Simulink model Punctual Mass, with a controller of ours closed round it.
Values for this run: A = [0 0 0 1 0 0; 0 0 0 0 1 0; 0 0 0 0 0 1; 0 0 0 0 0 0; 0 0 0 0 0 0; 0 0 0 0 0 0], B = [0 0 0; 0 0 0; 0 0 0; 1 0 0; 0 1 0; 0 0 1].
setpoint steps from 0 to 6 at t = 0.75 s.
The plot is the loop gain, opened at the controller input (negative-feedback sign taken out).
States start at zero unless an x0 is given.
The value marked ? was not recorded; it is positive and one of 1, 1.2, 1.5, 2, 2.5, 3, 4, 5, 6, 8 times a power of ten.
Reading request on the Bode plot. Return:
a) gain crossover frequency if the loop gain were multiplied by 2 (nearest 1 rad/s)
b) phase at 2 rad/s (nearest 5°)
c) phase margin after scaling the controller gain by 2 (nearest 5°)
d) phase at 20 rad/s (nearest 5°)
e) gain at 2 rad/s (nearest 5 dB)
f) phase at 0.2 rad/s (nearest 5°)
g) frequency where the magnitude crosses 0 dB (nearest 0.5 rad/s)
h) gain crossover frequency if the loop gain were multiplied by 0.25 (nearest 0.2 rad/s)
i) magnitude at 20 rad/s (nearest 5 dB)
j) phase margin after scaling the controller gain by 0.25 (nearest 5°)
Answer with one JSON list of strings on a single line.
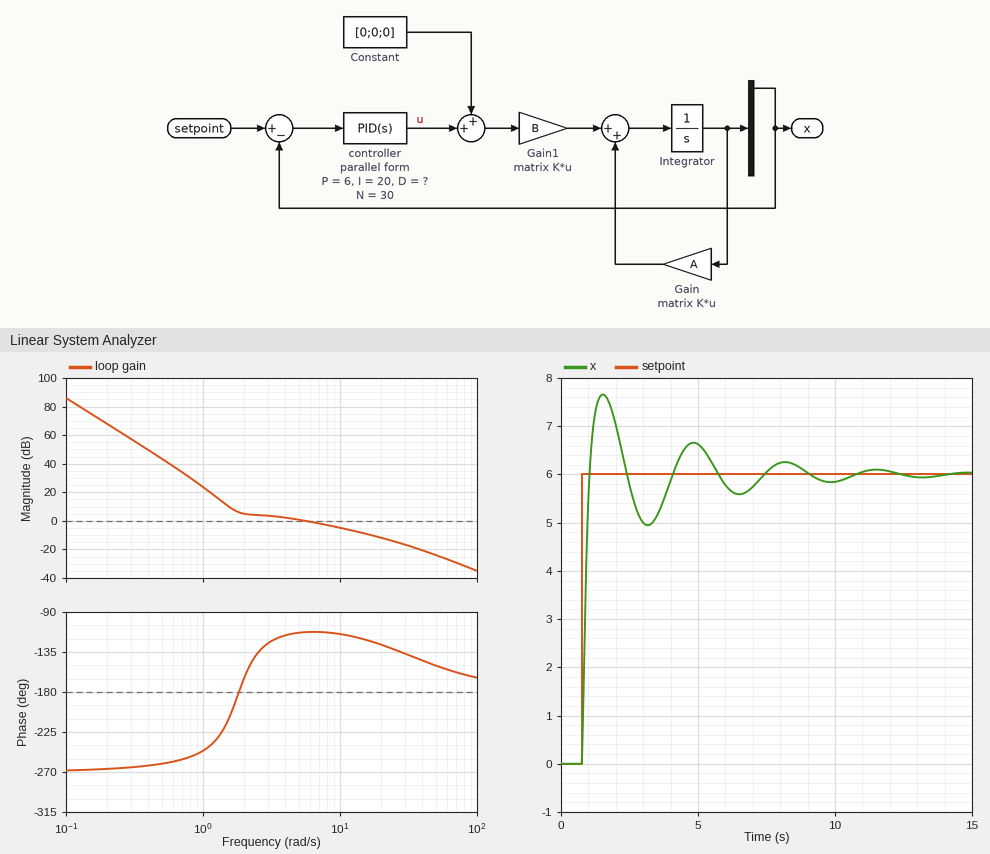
["11 rad/s", "-165°", "65°", "-125°", "5 dB", "-265°", "5.5 rad/s", "1.4 rad/s", "-10 dB", "-40°"]
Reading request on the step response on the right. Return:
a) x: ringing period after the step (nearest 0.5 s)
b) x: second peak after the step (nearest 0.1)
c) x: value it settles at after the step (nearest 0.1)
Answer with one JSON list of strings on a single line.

["3.5 s", "6.7", "6.0"]
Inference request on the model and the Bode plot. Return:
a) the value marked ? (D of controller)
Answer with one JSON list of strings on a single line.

["6"]
